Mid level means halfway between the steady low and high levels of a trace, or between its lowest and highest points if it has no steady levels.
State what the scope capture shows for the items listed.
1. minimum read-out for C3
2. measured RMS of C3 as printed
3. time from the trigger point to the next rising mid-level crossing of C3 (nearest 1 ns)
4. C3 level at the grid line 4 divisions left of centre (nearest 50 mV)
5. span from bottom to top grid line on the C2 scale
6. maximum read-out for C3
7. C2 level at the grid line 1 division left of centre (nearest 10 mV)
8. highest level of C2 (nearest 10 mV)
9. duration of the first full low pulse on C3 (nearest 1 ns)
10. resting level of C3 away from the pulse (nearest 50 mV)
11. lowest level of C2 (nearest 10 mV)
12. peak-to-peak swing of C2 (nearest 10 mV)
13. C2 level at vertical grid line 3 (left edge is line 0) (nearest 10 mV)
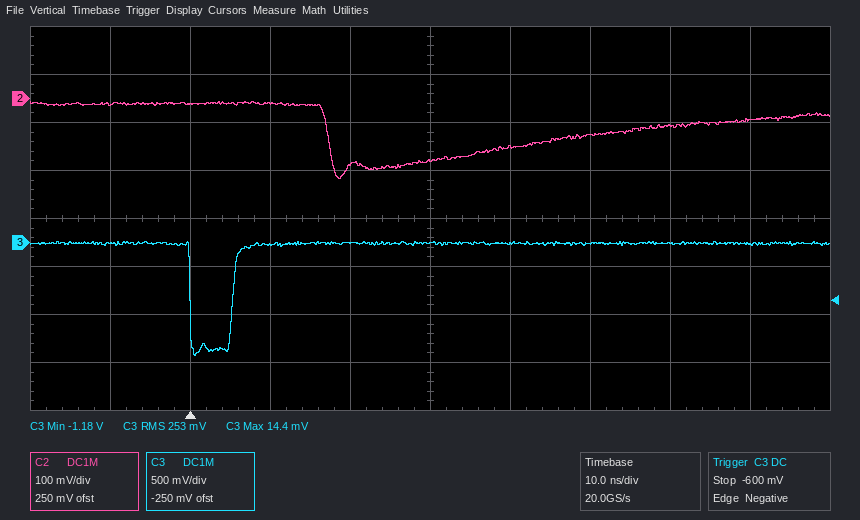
-1.18 V
253 mV
5 ns
0 mV
800 mV
14.4 mV
-140 mV
-10 mV
5 ns
0 mV
-170 mV
160 mV
-10 mV
